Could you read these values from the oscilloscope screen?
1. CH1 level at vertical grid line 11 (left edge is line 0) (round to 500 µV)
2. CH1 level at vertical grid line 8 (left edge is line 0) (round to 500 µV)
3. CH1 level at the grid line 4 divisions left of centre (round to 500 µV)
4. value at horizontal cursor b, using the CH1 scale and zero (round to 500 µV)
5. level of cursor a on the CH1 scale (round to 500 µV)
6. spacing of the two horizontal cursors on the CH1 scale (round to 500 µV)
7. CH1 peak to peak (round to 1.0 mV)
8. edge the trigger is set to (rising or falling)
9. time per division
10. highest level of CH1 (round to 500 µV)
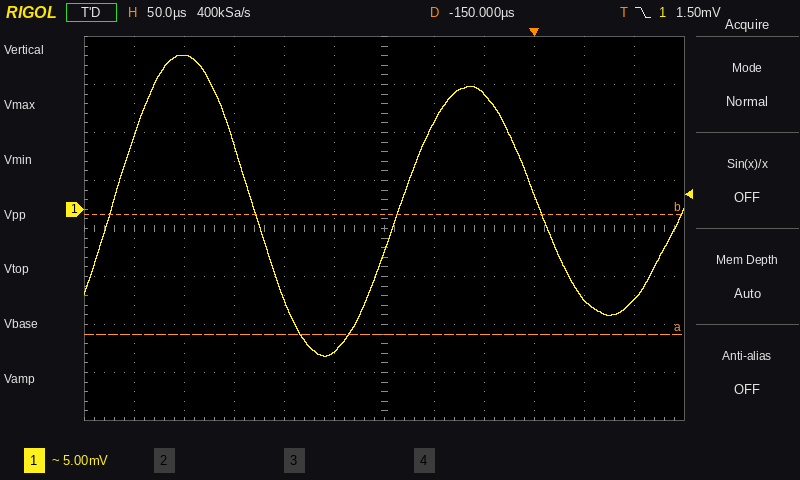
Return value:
-9.5 mV
12.0 mV
16.0 mV
-500 µV
-13.0 mV
12.5 mV
31.0 mV
falling
50 µs
16.0 mV
